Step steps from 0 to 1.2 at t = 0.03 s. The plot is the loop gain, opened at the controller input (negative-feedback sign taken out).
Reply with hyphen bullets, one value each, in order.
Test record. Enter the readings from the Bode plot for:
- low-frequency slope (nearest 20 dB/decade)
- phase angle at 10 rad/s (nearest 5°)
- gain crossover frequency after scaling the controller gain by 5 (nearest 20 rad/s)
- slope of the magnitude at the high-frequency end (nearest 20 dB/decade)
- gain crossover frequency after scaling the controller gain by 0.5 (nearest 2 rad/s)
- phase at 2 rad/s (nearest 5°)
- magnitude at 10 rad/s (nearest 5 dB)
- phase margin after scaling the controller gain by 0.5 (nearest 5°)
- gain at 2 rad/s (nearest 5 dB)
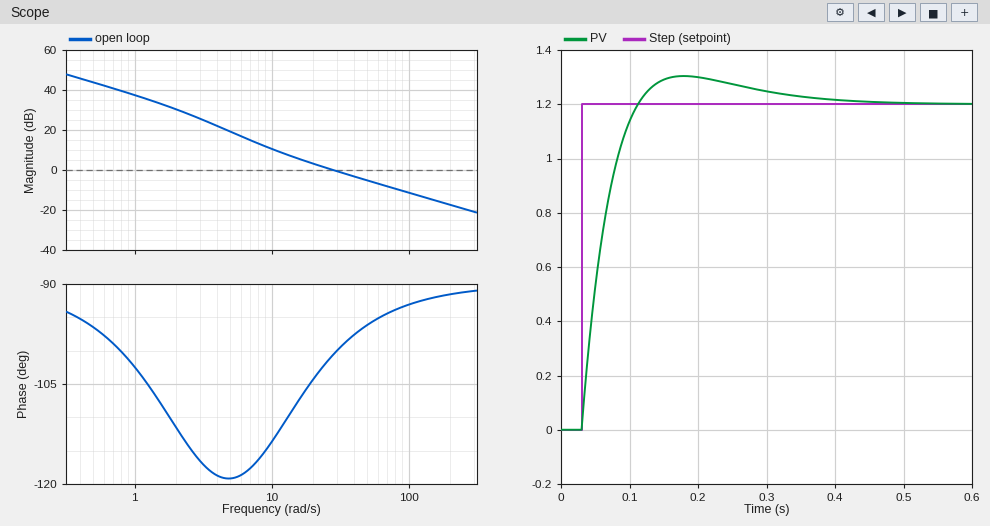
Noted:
- -20 dB/decade
- -115°
- 140 rad/s
- -20 dB/decade
- 16 rad/s
- -110°
- 10 dB
- 70°
- 30 dB
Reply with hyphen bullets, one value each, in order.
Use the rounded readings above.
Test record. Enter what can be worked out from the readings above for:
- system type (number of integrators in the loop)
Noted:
- 1
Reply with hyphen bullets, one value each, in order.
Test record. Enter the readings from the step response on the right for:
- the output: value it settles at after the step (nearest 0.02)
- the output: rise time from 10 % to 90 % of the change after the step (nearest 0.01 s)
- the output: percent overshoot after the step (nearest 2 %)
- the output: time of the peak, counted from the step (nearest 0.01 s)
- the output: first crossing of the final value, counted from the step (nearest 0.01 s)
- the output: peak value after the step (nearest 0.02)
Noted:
- 1.20
- 0.06 s
- 8 %
- 0.15 s
- 0.08 s
- 1.30
